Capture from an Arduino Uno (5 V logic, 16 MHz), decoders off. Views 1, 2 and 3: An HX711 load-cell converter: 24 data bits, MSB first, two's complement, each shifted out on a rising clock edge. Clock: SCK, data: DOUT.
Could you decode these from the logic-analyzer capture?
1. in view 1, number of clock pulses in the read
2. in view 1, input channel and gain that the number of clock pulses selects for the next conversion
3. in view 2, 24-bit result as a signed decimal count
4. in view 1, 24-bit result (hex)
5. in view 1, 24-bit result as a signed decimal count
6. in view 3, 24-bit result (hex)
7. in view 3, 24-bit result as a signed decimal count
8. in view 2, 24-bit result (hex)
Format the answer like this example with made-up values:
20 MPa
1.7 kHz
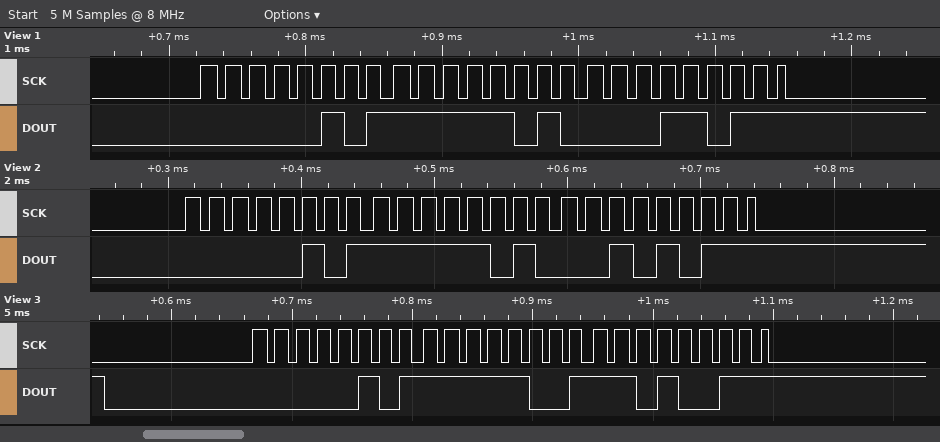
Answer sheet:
25
channel A, gain 128
391723
0x05FA1B
391707
0x05F9D3
391635
0x05FA2B
